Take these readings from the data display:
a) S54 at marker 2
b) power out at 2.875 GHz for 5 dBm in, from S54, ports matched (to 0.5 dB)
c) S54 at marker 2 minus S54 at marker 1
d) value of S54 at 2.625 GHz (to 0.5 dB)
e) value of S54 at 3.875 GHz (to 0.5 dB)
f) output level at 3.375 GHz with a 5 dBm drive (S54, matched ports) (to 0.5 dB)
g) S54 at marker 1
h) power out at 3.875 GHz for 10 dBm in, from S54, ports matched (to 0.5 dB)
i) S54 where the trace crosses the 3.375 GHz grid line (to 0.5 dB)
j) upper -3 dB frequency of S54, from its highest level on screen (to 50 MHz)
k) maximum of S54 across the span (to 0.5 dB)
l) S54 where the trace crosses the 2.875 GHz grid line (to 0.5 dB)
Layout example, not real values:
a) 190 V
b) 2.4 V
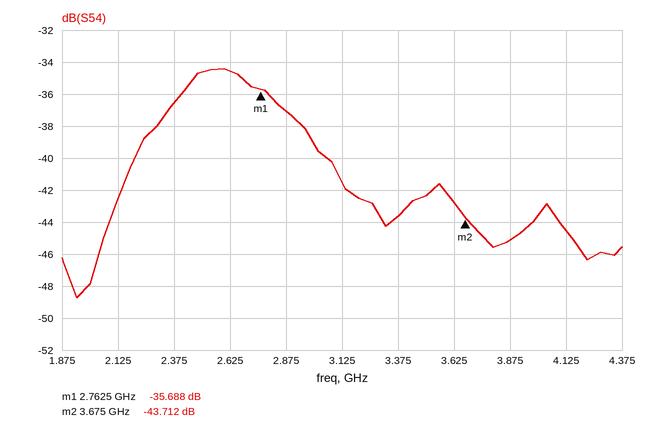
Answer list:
a) -43.712 dB
b) -32.0 dBm
c) -8.024 dB
d) -34.5 dB
e) -45.0 dB
f) -38.5 dBm
g) -35.688 dB
h) -35.0 dBm
i) -43.5 dB
j) 2.90 GHz
k) -34.5 dB
l) -37.0 dB
